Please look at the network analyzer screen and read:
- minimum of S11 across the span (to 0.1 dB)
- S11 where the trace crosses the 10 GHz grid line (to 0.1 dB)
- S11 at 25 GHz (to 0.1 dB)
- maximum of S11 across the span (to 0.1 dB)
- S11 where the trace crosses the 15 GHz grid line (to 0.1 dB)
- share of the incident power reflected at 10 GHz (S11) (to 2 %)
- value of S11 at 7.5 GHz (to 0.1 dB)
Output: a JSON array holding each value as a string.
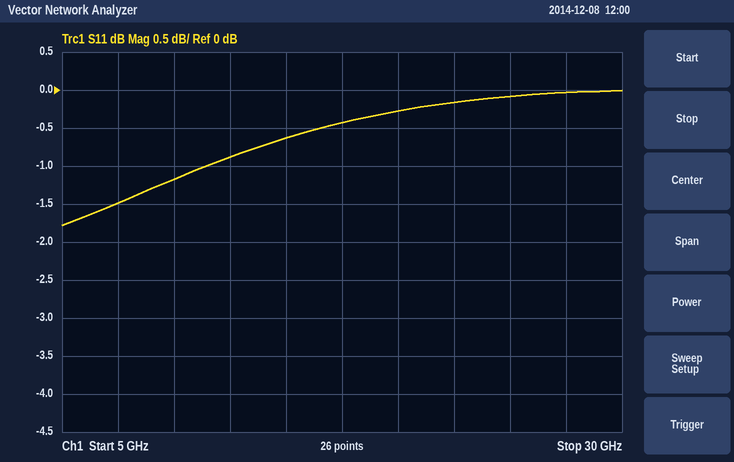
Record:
["-1.8 dB", "-1.2 dB", "-0.1 dB", "0.0 dB", "-0.6 dB", "76 %", "-1.5 dB"]
